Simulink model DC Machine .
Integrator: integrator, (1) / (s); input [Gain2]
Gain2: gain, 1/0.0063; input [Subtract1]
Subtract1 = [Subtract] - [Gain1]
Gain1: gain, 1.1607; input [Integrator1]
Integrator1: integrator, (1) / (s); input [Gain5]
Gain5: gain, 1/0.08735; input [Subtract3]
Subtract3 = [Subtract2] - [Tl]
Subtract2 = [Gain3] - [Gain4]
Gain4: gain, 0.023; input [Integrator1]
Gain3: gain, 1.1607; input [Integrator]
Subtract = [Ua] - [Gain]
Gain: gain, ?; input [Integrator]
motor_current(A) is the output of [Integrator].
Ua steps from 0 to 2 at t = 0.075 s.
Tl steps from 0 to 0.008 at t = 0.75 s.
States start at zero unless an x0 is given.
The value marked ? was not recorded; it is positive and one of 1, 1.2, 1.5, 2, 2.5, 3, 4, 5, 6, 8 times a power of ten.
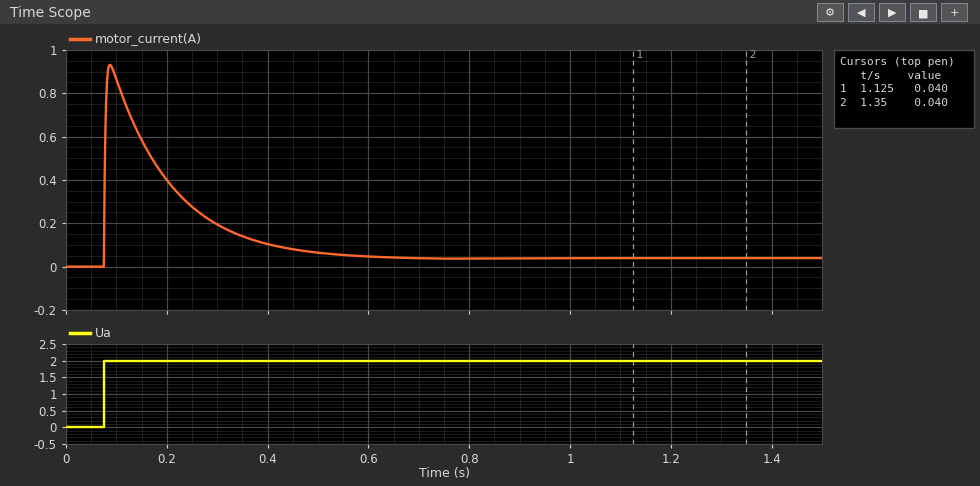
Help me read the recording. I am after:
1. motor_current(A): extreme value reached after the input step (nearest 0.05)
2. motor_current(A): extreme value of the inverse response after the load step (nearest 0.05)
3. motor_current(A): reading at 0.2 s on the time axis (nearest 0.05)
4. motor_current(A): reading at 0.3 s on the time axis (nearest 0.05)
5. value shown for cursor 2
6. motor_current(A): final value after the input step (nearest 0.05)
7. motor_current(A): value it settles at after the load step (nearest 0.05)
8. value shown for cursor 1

0.95
0.05
0.40
0.20
0.040
0.05
0.05
0.040
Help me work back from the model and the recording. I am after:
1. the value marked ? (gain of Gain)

2
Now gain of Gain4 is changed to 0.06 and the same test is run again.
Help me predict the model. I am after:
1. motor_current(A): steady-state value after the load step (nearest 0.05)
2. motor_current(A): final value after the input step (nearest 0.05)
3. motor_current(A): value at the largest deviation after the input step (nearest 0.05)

0.10
0.10
0.95
